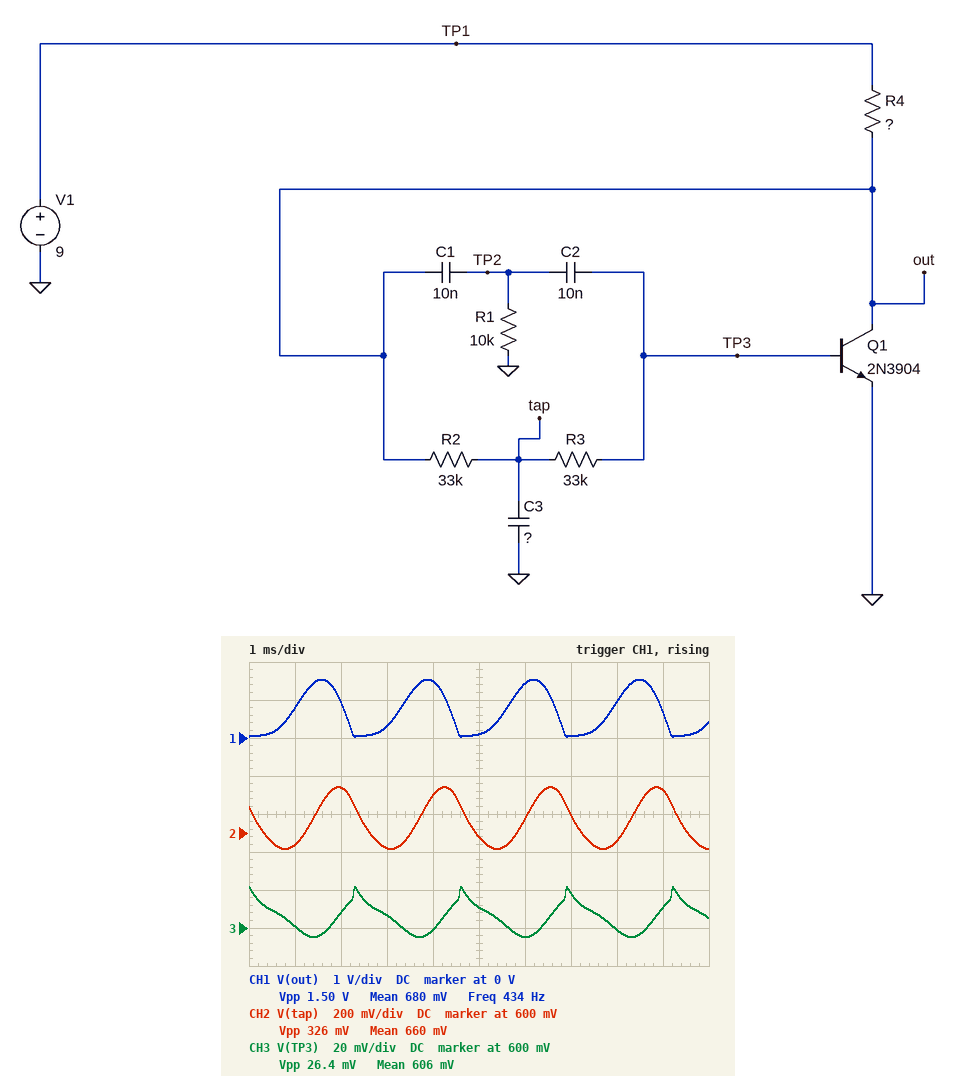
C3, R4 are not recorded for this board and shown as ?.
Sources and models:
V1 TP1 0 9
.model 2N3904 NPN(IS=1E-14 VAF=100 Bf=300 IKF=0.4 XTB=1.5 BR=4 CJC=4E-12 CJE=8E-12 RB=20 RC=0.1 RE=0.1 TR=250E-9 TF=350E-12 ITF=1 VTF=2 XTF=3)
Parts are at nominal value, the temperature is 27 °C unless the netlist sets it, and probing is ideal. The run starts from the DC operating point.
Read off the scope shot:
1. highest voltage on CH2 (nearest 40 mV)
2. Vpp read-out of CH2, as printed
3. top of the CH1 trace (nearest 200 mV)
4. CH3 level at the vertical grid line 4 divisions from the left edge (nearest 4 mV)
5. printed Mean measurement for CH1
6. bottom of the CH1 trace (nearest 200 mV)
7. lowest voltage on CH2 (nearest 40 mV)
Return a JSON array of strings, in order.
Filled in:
["840 mV", "326 mV", "1.6 V", "600 mV", "680 mV", "0 V", "520 mV"]
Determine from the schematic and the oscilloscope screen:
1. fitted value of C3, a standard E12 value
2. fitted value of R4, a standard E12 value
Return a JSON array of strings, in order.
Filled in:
["47 nF", "56 kΩ"]
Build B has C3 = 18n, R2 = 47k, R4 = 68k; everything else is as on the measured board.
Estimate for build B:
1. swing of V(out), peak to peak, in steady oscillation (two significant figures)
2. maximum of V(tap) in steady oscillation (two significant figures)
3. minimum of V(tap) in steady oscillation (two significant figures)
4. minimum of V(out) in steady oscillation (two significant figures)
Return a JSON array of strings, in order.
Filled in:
["1.3 V", "810 mV", "470 mV", "47 mV"]
